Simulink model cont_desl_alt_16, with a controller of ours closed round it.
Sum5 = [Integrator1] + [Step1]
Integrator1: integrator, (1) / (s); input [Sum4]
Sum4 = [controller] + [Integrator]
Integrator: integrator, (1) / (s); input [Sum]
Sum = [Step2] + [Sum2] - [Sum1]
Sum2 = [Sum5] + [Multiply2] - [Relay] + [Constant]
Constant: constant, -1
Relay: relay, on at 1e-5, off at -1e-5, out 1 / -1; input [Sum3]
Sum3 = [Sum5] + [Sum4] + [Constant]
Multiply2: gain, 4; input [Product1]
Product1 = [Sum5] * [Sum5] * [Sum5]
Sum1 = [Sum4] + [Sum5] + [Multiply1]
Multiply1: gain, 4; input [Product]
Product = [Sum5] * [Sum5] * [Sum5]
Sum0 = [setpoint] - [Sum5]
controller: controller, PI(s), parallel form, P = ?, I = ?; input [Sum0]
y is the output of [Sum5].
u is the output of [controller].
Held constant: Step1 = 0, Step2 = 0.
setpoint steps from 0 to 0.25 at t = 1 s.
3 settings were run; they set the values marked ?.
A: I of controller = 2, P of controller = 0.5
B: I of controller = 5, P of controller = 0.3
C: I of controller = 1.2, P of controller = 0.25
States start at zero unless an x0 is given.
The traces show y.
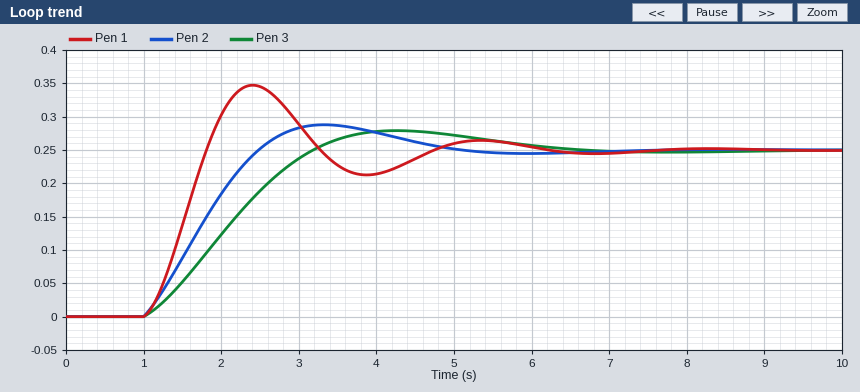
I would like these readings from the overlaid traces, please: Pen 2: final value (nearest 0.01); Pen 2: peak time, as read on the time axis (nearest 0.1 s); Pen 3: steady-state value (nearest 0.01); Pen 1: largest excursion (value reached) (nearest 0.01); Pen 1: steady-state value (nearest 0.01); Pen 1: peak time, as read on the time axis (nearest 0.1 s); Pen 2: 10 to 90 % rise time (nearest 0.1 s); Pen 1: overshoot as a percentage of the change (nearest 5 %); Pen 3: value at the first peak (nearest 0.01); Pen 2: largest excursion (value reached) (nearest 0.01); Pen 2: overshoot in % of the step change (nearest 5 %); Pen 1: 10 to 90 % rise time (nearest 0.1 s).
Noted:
0.25
3.3 s
0.25
0.35
0.25
2.4 s
1.1 s
40 %
0.28
0.29
15 %
0.6 s
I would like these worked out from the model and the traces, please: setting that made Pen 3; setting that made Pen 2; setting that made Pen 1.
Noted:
C
A
B
